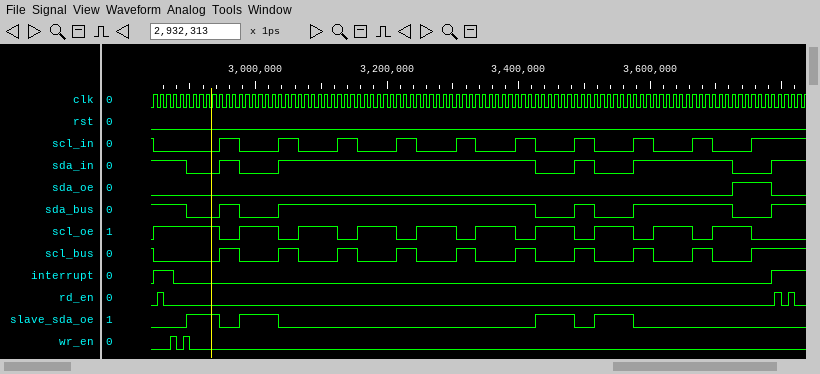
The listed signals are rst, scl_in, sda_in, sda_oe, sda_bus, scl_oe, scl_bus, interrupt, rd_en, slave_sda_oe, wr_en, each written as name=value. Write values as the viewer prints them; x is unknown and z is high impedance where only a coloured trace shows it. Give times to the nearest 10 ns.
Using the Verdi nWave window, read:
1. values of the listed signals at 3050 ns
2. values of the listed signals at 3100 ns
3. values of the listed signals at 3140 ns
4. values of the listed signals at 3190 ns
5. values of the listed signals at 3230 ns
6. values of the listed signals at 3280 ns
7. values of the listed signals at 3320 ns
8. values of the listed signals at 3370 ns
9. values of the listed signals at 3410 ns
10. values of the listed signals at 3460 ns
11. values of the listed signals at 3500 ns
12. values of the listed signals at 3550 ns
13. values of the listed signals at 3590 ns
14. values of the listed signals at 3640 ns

rst=0, scl_in=1, sda_in=1, sda_oe=0, sda_bus=1, scl_oe=0, scl_bus=1, interrupt=0, rd_en=0, slave_sda_oe=0, wr_en=0
rst=0, scl_in=0, sda_in=1, sda_oe=0, sda_bus=1, scl_oe=1, scl_bus=0, interrupt=0, rd_en=0, slave_sda_oe=0, wr_en=0
rst=0, scl_in=1, sda_in=1, sda_oe=0, sda_bus=1, scl_oe=0, scl_bus=1, interrupt=0, rd_en=0, slave_sda_oe=0, wr_en=0
rst=0, scl_in=0, sda_in=1, sda_oe=0, sda_bus=1, scl_oe=1, scl_bus=0, interrupt=0, rd_en=0, slave_sda_oe=0, wr_en=0
rst=0, scl_in=1, sda_in=1, sda_oe=0, sda_bus=1, scl_oe=0, scl_bus=1, interrupt=0, rd_en=0, slave_sda_oe=0, wr_en=0
rst=0, scl_in=0, sda_in=1, sda_oe=0, sda_bus=1, scl_oe=1, scl_bus=0, interrupt=0, rd_en=0, slave_sda_oe=0, wr_en=0
rst=0, scl_in=1, sda_in=1, sda_oe=0, sda_bus=1, scl_oe=0, scl_bus=1, interrupt=0, rd_en=0, slave_sda_oe=0, wr_en=0
rst=0, scl_in=0, sda_in=1, sda_oe=0, sda_bus=1, scl_oe=1, scl_bus=0, interrupt=0, rd_en=0, slave_sda_oe=0, wr_en=0
rst=0, scl_in=1, sda_in=1, sda_oe=0, sda_bus=1, scl_oe=0, scl_bus=1, interrupt=0, rd_en=0, slave_sda_oe=0, wr_en=0
rst=0, scl_in=0, sda_in=0, sda_oe=0, sda_bus=0, scl_oe=1, scl_bus=0, interrupt=0, rd_en=0, slave_sda_oe=1, wr_en=0
rst=0, scl_in=1, sda_in=1, sda_oe=0, sda_bus=1, scl_oe=0, scl_bus=1, interrupt=0, rd_en=0, slave_sda_oe=0, wr_en=0
rst=0, scl_in=0, sda_in=0, sda_oe=0, sda_bus=0, scl_oe=1, scl_bus=0, interrupt=0, rd_en=0, slave_sda_oe=1, wr_en=0
rst=0, scl_in=1, sda_in=1, sda_oe=0, sda_bus=1, scl_oe=0, scl_bus=1, interrupt=0, rd_en=0, slave_sda_oe=0, wr_en=0
rst=0, scl_in=0, sda_in=1, sda_oe=0, sda_bus=1, scl_oe=1, scl_bus=0, interrupt=0, rd_en=0, slave_sda_oe=0, wr_en=0
